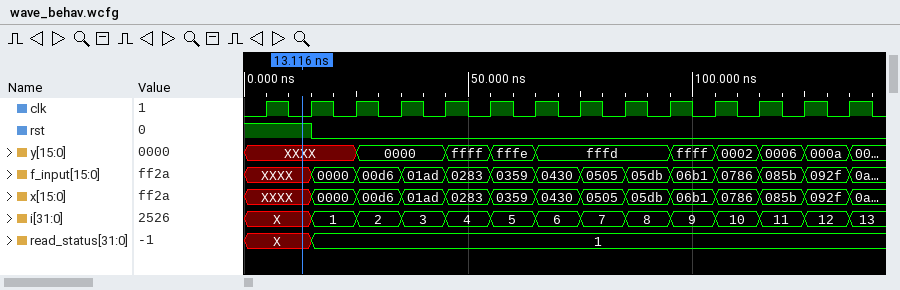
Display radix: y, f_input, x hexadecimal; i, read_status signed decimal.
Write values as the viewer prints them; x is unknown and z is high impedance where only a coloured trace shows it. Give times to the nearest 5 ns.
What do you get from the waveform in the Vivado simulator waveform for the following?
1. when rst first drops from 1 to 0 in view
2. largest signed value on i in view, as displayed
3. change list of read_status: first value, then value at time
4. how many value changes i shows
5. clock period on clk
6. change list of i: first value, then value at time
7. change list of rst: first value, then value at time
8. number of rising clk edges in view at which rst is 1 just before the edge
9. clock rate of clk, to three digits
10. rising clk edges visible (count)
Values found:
15 ns
13
X, 1 at 15 ns
13
10 ns
X, 1 at 15 ns, 2 at 25 ns, 3 at 35 ns, 4 at 45 ns, 5 at 55 ns, 6 at 65 ns, 7 at 75 ns, 8 at 85 ns, 9 at 95 ns, 10 at 105 ns, 11 at 115 ns, 12 at 125 ns, 13 at 135 ns
1, 0 at 15 ns
2
100 MHz
14
